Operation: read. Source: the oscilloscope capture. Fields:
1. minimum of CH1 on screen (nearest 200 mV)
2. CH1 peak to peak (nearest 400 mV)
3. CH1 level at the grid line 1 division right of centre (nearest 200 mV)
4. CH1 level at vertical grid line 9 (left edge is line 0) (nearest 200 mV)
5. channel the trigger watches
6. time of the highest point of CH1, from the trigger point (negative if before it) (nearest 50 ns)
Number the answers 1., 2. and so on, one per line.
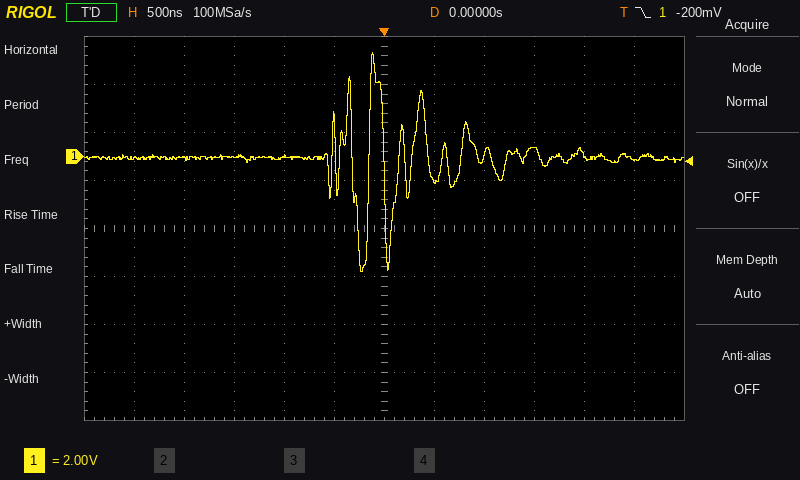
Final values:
1. -4.8 V
2. 9.2 V
3. -1.0 V
4. 400 mV
5. CH1
6. -100 ns
